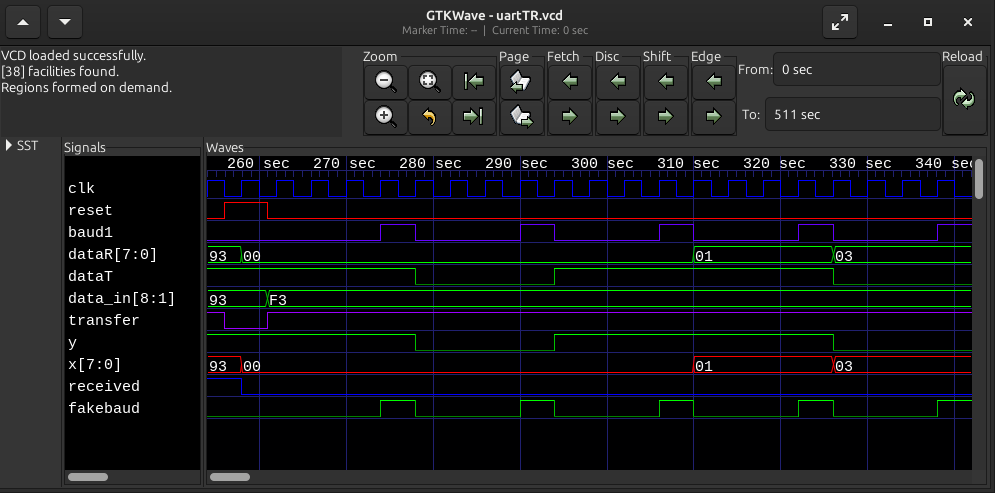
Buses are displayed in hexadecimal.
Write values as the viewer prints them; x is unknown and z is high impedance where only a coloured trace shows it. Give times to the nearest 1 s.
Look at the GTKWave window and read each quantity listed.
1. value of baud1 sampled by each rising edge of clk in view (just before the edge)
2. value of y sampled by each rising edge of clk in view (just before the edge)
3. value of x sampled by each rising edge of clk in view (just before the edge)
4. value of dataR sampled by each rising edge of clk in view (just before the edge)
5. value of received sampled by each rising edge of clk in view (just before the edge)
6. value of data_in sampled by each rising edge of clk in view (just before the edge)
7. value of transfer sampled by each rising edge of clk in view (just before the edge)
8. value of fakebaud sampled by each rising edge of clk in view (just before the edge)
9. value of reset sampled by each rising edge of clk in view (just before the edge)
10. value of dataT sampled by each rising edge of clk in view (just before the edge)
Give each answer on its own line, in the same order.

0 0 0 0 0 1 0 0 0 1 0 0 0 1 0 0 0 1 0 0 0
1 1 1 1 1 1 0 0 0 0 1 1 1 1 1 1 1 1 0 0 0
93, 00, 00, 00, 00, 00, 00, 00, 00, 00, 00, 00, 00, 00, 01, 01, 01, 01, 03, 03, 03
93, 00, 00, 00, 00, 00, 00, 00, 00, 00, 00, 00, 00, 00, 01, 01, 01, 01, 03, 03, 03
1 0 0 0 0 0 0 0 0 0 0 0 0 0 0 0 0 0 0 0 0
93, F3, F3, F3, F3, F3, F3, F3, F3, F3, F3, F3, F3, F3, F3, F3, F3, F3, F3, F3, F3
0 1 1 1 1 1 1 1 1 1 1 1 1 1 1 1 1 1 1 1 1
0 0 0 0 0 1 0 0 0 1 0 0 0 1 0 0 0 1 0 0 0
1 0 0 0 0 0 0 0 0 0 0 0 0 0 0 0 0 0 0 0 0
1 1 1 1 1 1 0 0 0 0 1 1 1 1 1 1 1 1 0 0 0
